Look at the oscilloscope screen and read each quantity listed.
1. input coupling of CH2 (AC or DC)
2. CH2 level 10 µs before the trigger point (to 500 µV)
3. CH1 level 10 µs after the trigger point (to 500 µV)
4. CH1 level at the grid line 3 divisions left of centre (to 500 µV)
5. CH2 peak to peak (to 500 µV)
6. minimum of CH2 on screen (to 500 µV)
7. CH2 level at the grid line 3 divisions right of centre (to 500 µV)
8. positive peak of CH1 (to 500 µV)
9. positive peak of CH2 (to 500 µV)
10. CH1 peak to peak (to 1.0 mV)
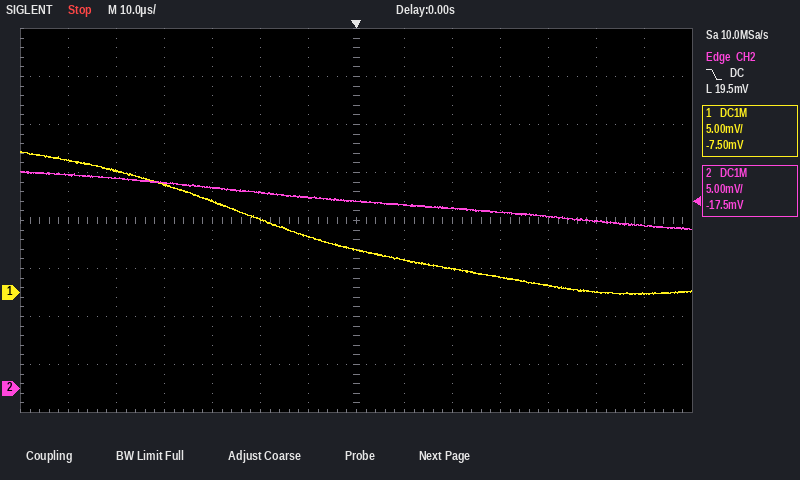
DC
20.0 mV
3.5 mV
9.5 mV
6.0 mV
16.5 mV
18.5 mV
14.5 mV
22.5 mV
15.0 mV
